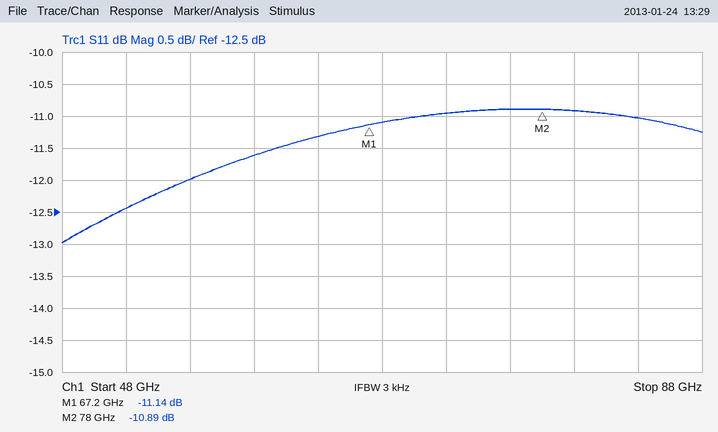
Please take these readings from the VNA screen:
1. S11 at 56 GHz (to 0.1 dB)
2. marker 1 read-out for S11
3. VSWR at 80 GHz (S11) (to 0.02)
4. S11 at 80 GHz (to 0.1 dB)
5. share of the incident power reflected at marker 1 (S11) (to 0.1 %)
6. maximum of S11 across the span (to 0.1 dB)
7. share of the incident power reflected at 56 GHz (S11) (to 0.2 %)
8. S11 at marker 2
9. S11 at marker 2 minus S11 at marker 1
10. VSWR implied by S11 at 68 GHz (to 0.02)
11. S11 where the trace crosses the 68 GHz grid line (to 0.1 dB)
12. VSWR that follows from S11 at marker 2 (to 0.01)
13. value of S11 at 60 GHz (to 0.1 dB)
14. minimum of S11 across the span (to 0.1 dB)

-12.0 dB
-11.14 dB
1.80
-10.9 dB
7.7 %
-10.9 dB
6.4 %
-10.89 dB
0.25 dB
1.78
-11.1 dB
1.80
-11.6 dB
-13.0 dB
